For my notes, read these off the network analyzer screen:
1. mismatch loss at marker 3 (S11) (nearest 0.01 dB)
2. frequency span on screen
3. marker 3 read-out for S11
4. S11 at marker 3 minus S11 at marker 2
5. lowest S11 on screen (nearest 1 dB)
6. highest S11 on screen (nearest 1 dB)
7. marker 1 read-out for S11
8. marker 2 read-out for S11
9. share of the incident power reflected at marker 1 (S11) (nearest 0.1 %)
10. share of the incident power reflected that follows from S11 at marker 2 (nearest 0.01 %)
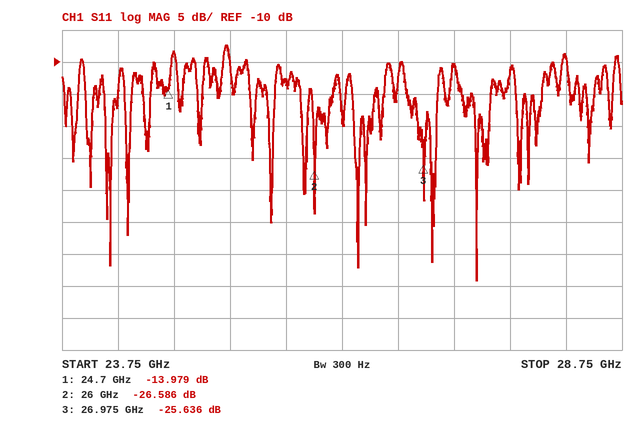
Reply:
0.01 dB
5 GHz
-25.636 dB
0.950 dB
-44 dB
-7 dB
-13.979 dB
-26.586 dB
4.0 %
0.22 %
